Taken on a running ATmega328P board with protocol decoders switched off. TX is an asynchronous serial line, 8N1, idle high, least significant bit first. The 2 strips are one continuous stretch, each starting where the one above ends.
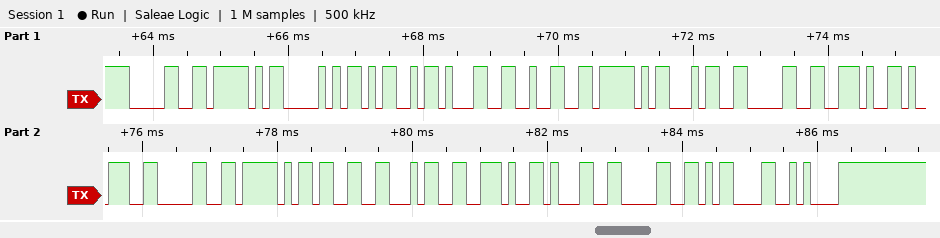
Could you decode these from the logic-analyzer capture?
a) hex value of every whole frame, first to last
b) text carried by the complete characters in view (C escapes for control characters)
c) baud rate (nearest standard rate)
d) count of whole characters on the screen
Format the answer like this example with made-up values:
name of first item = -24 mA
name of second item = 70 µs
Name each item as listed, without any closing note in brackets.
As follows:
hex value of every whole frame, first to last = 30 5F 50 4D 31 32 5F 34 30 2E 39 30 5F 33 34 2E 31 30 0D 0A
text carried by the complete characters in view = "0_PM12_40.90_34.10\r\n"
baud rate = 9600 baud
count of whole characters on the screen = 20
